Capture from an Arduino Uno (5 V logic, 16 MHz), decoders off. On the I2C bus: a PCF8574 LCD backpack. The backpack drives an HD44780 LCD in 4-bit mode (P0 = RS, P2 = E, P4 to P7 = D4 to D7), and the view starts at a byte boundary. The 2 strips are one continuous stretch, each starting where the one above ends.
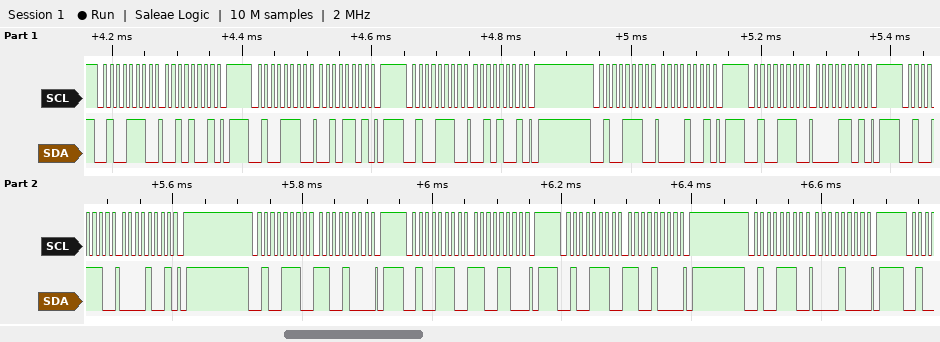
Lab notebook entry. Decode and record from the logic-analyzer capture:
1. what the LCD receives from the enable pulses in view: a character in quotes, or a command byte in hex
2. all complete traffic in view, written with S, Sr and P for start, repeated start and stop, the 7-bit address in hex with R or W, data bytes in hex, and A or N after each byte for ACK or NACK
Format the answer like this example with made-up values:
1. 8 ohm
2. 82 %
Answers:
1. ' '
2. S 27W A 29 A P S 27W A 2D A P S 27W A 29 A P S 27W A 09 A P S 27W A 0D A P S 27W A 09 A P S 27W A C8 A P S 27W A CC A P S 27W A C8 A P S 27W A 08 A P
